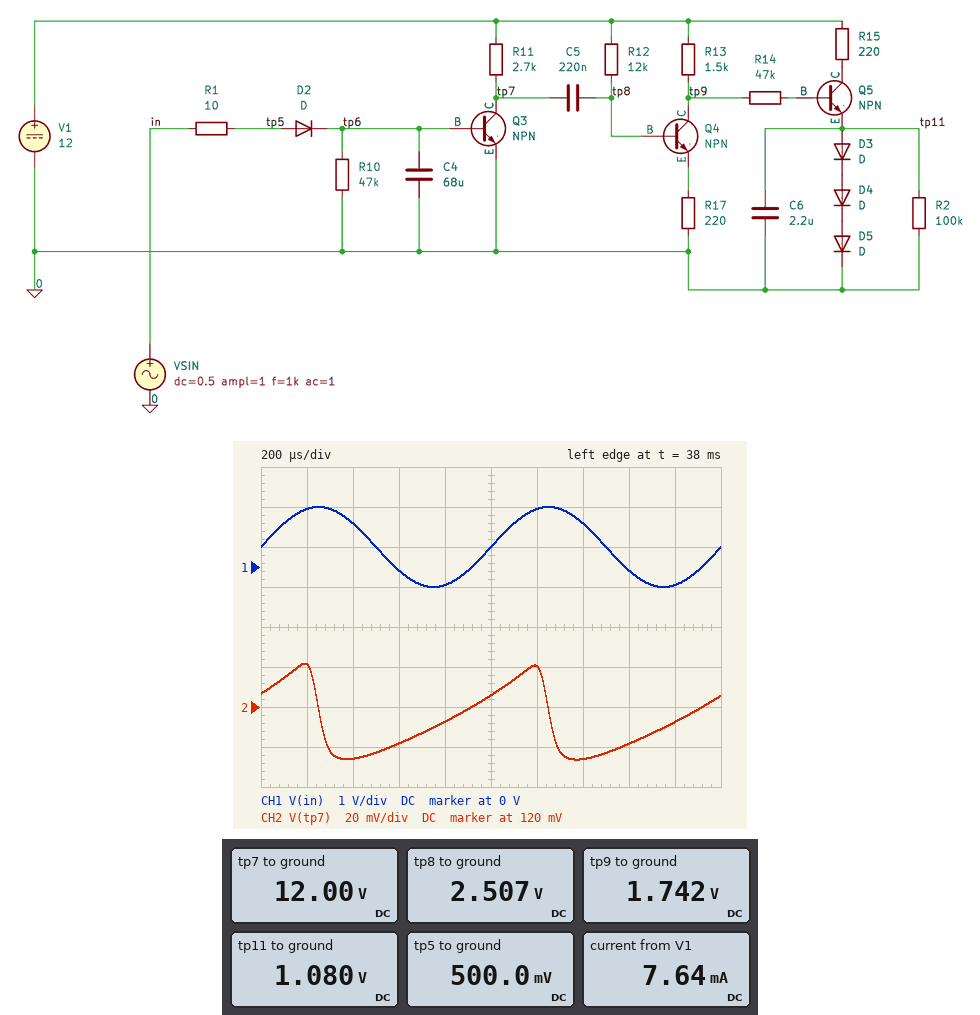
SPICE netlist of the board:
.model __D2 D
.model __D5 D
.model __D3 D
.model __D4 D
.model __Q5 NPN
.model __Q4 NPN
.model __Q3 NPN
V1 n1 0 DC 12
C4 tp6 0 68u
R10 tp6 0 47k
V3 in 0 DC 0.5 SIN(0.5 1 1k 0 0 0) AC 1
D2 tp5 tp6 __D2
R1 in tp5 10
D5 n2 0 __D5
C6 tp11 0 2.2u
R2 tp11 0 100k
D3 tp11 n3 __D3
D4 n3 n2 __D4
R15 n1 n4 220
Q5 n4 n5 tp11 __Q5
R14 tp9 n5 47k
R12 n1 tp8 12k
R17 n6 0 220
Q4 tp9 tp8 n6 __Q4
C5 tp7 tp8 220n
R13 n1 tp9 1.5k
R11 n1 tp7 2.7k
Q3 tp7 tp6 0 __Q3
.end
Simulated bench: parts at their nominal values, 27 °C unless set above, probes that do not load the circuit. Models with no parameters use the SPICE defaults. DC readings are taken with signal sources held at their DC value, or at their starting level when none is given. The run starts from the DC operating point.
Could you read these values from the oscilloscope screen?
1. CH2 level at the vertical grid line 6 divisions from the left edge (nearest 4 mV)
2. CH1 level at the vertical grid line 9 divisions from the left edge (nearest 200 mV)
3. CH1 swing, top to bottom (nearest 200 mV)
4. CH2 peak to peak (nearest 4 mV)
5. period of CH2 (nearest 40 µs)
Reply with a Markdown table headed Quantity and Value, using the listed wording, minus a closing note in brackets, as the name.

| Quantity | Value |
|---|---|
| CH2 level at the vertical grid line 6 divisions from the left edge | 140 mV |
| CH1 level at the vertical grid line 9 divisions from the left edge | -400 mV |
| CH1 swing, top to bottom | 2.0 V |
| CH2 peak to peak | 48 mV |
| period of CH2 | 1.00 ms |
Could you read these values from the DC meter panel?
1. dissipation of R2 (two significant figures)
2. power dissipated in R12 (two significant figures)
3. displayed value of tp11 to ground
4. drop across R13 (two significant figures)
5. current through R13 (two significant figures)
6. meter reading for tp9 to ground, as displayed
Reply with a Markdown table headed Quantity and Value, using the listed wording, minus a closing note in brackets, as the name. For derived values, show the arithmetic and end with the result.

| Quantity | Value |
|---|---|
| dissipation of R2 | (1.08 V)^2 / 100 kΩ = 12 µW |
| power dissipated in R12 | (12 V - 2.507 V)^2 / 12 kΩ = 7.5 mW |
| displayed value of tp11 to ground | 1.080 V |
| drop across R13 | 12 V - 1.742 V = 10 V |
| current through R13 | (12 V - 1.742 V) / 1.5 kΩ = 6.8 mA |
| meter reading for tp9 to ground, as displayed | 1.742 V |
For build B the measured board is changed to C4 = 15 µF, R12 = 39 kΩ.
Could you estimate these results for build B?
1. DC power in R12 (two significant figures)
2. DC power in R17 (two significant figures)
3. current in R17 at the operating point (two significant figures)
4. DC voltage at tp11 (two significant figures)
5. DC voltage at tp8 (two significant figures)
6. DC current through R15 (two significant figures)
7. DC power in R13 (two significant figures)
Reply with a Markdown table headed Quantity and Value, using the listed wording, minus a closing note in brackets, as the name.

| Quantity | Value |
|---|---|
| DC power in R12 | 2.4 mW |
| DC power in R17 | 11 mW |
| current in R17 at the operating point | 7.1 mA |
| DC voltage at tp11 | 1.0 V |
| DC voltage at tp8 | 2.4 V |
| DC current through R15 | 10 µA |
| DC power in R13 | 71 mW |
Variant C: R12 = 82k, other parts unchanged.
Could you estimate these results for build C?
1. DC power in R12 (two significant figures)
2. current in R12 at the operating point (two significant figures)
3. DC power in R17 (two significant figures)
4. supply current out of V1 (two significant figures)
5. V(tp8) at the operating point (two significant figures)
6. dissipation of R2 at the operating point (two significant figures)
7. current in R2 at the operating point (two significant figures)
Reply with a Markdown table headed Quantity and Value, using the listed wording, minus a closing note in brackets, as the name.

| Quantity | Value |
|---|---|
| DC power in R12 | 1.1 mW |
| current in R12 at the operating point | 120 µA |
| DC power in R17 | 11 mW |
| supply current out of V1 | 7.0 mA |
| V(tp8) at the operating point | 2.4 V |
| dissipation of R2 at the operating point | 10 µW |
| current in R2 at the operating point | 10 µA |
